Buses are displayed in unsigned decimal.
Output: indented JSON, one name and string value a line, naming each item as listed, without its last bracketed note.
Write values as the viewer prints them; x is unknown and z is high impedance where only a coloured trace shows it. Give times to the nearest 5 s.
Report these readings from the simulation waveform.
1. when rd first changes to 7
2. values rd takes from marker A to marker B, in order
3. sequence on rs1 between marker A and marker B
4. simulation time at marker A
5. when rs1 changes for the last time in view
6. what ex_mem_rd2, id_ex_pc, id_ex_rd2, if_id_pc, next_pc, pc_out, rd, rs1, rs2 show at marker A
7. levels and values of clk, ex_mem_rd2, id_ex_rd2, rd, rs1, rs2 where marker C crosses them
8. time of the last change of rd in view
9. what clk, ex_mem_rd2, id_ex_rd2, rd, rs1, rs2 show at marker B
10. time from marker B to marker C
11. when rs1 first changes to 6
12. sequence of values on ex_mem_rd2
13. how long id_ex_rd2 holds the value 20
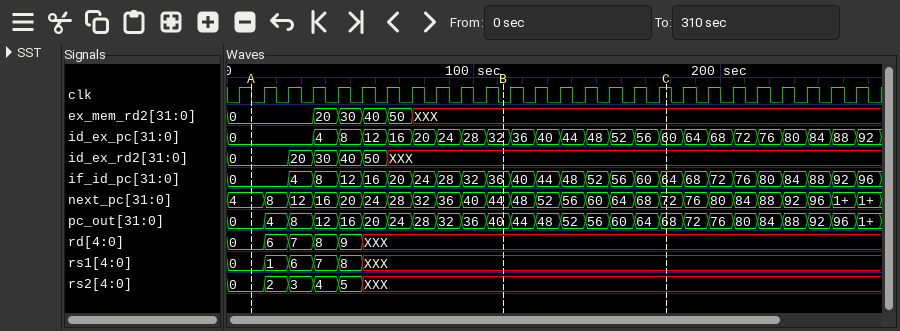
{
  "when rd first changes to 7": "25 s",
  "values rd takes from marker A to marker B, in order": "0, 6, 7, 8, 9, XXX",
  "sequence on rs1 between marker A and marker B": "0, 1, 6, 7, 8, XXX",
  "simulation time at marker A": "10 s",
  "when rs1 changes for the last time in view": "55 s",
  "what ex_mem_rd2, id_ex_pc, id_ex_rd2, if_id_pc, next_pc, pc_out, rd, rs1, rs2 show at marker A": "ex_mem_rd2=0, id_ex_pc=0, id_ex_rd2=0, if_id_pc=0, next_pc=4, pc_out=0, rd=0, rs1=0, rs2=0",
  "levels and values of clk, ex_mem_rd2, id_ex_rd2, rd, rs1, rs2 where marker C crosses them": "clk=1, ex_mem_rd2=XXX, id_ex_rd2=XXX, rd=XXX, rs1=XXX, rs2=XXX",
  "time of the last change of rd in view": "55 s",
  "what clk, ex_mem_rd2, id_ex_rd2, rd, rs1, rs2 show at marker B": "clk=0, ex_mem_rd2=XXX, id_ex_rd2=XXX, rd=XXX, rs1=XXX, rs2=XXX",
  "time from marker B to marker C": "65 s",
  "when rs1 first changes to 6": "25 s",
  "sequence of values on ex_mem_rd2": "0, 20, 30, 40, 50, XXX",
  "how long id_ex_rd2 holds the value 20": "10 s"
}
